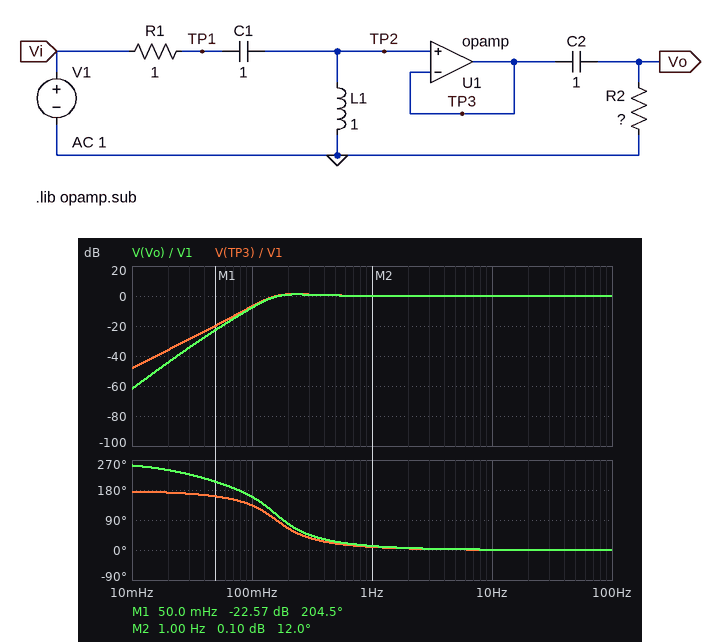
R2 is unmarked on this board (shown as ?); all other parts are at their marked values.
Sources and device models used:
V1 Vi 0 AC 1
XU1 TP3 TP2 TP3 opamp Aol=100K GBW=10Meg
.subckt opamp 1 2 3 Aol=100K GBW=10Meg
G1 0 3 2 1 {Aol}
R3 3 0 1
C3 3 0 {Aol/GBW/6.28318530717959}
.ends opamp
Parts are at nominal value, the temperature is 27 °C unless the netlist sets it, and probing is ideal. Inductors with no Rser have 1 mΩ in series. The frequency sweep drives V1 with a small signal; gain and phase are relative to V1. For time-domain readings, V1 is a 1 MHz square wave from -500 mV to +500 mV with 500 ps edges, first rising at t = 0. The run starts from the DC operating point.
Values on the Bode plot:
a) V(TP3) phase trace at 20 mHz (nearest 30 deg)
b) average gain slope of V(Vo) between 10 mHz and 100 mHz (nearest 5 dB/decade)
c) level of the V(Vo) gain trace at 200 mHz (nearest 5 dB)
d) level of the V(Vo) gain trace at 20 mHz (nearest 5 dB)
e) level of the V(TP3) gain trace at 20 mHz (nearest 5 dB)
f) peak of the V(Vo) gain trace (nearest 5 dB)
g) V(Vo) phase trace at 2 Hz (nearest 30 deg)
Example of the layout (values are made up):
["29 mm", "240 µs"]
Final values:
["180 deg", "55 dB/decade", "0 dB", "-45 dB", "-35 dB", "0 dB", "0 deg"]
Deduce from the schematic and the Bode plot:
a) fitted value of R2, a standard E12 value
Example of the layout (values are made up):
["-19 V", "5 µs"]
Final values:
["3.3 Ω"]
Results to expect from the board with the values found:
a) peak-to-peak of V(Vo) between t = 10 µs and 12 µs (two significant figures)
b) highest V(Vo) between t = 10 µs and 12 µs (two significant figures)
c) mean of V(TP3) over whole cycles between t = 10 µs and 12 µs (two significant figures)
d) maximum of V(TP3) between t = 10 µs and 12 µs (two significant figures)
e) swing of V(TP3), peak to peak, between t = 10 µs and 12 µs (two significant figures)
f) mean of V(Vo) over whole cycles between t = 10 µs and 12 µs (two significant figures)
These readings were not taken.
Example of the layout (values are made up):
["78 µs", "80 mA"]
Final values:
["1.0 V", "1.0 V", "500 mV", "1.0 V", "1.0 V", "500 mV"]
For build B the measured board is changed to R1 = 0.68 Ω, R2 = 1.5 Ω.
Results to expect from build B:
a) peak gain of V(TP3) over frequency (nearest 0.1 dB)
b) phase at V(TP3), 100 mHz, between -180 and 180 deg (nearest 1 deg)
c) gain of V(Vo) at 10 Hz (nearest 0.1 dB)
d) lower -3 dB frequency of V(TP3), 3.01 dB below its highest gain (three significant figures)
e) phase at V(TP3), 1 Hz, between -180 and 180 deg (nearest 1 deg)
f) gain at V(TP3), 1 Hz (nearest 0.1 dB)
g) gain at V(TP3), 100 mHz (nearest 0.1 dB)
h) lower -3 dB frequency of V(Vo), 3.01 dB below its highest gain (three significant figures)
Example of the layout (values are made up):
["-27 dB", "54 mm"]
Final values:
["3.9 dB", "145 deg", "0 dB", "134 mHz", "6 deg", "0.2 dB", "-5.5 dB", "140 mHz"]
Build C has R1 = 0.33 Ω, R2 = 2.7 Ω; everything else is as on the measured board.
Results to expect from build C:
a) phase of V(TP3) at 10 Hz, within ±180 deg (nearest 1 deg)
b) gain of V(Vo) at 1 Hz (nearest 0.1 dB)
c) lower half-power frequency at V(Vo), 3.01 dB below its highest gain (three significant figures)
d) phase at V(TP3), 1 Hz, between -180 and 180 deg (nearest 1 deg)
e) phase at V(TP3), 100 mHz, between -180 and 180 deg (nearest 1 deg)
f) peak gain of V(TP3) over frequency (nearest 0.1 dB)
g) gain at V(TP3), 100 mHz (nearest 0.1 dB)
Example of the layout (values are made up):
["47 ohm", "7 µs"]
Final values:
["0 deg", "0.2 dB", "142 mHz", "3 deg", "161 deg", "9.7 dB", "-4.2 dB"]
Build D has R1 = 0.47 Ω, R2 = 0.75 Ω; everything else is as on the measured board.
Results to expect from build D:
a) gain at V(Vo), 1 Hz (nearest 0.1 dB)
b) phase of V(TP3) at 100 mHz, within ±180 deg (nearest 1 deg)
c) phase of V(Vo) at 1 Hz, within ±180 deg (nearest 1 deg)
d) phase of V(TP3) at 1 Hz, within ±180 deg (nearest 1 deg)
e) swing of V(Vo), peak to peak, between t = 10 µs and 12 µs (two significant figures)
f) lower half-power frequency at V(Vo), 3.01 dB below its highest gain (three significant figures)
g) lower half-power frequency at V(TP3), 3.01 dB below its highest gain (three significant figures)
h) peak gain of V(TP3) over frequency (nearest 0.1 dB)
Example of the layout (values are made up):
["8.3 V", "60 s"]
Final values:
["0 dB", "154 deg", "16 deg", "4 deg", "1.0 V", "143 mHz", "137 mHz", "6.8 dB"]
